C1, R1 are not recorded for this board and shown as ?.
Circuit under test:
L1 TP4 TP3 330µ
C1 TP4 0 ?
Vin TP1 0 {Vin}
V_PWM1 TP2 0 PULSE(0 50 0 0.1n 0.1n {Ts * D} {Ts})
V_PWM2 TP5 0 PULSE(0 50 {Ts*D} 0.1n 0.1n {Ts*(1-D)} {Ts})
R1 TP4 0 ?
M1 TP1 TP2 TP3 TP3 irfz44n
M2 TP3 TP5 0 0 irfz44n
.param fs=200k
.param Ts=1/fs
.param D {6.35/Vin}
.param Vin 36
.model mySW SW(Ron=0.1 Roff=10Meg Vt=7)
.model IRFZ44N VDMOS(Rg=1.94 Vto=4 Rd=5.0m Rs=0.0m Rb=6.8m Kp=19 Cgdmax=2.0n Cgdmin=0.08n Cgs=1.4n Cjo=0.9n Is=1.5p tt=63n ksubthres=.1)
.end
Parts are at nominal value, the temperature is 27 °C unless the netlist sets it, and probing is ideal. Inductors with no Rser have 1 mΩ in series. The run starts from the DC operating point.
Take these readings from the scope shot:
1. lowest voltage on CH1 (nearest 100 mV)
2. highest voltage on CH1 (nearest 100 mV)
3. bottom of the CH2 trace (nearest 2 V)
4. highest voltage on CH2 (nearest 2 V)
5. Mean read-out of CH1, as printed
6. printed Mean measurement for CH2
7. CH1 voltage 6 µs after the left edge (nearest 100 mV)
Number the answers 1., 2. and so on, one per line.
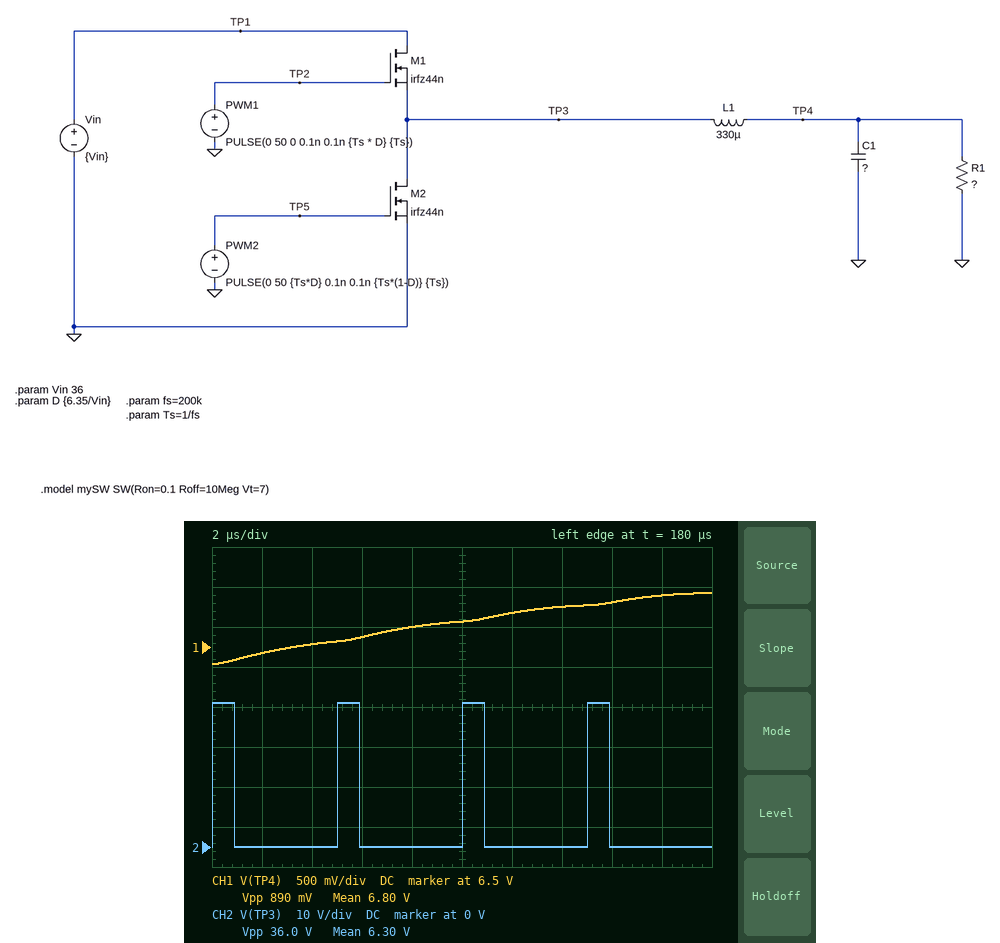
1. 6.3 V
2. 7.2 V
3. 0 V
4. 36 V
5. 6.80 V
6. 6.30 V
7. 6.6 V
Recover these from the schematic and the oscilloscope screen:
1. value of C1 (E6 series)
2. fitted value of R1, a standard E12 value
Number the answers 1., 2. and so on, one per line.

1. 1.5 µF
2. 39 Ω
